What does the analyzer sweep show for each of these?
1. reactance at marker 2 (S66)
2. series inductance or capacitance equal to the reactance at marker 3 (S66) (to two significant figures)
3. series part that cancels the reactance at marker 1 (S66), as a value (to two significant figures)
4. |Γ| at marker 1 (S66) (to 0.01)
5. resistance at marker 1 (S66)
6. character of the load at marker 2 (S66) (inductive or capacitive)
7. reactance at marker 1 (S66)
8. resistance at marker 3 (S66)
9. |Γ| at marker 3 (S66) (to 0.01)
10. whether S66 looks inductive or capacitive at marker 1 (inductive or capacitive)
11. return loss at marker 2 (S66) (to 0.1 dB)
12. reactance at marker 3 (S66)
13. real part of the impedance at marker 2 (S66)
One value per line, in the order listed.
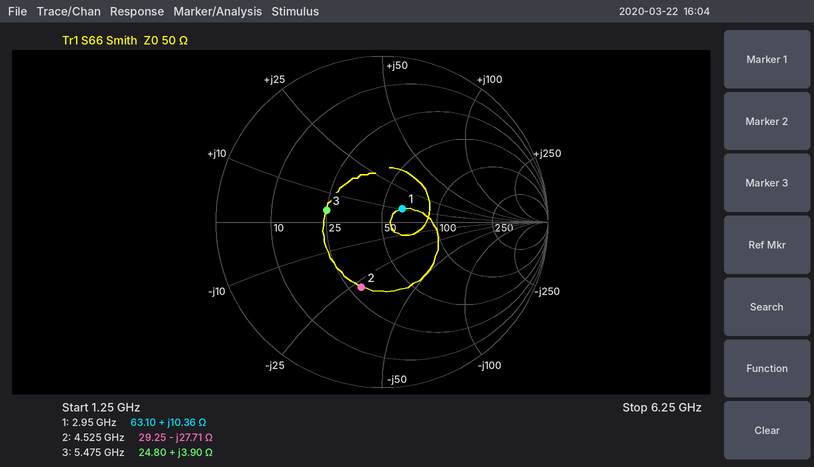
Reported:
-27.71 Ω
110 pH
5.2 pF
0.15
63.10 Ω
capacitive
+10.36 Ω
24.80 Ω
0.34
inductive
7.7 dB
+3.90 Ω
29.25 Ω
